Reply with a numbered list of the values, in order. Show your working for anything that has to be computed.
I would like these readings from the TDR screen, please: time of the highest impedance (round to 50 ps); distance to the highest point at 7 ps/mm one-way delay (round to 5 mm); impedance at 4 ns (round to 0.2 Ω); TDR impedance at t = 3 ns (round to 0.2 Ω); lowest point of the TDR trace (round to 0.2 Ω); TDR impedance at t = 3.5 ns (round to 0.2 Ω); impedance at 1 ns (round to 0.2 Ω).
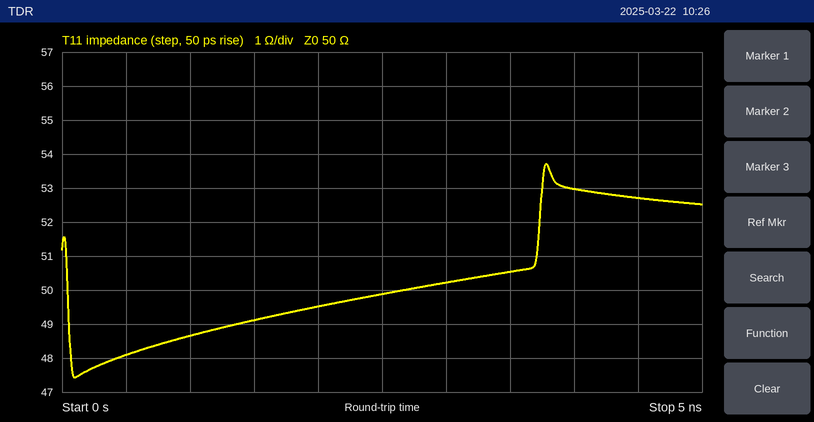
1. 3.80 ns
2. 3.80 ns / 2 / 7 ps/mm ≈ 271 mm, so 270 mm to the nearest 5 mm
3. 53.0 Ω
4. 50.2 Ω
5. 47.4 Ω
6. 50.6 Ω
7. 48.6 Ω
